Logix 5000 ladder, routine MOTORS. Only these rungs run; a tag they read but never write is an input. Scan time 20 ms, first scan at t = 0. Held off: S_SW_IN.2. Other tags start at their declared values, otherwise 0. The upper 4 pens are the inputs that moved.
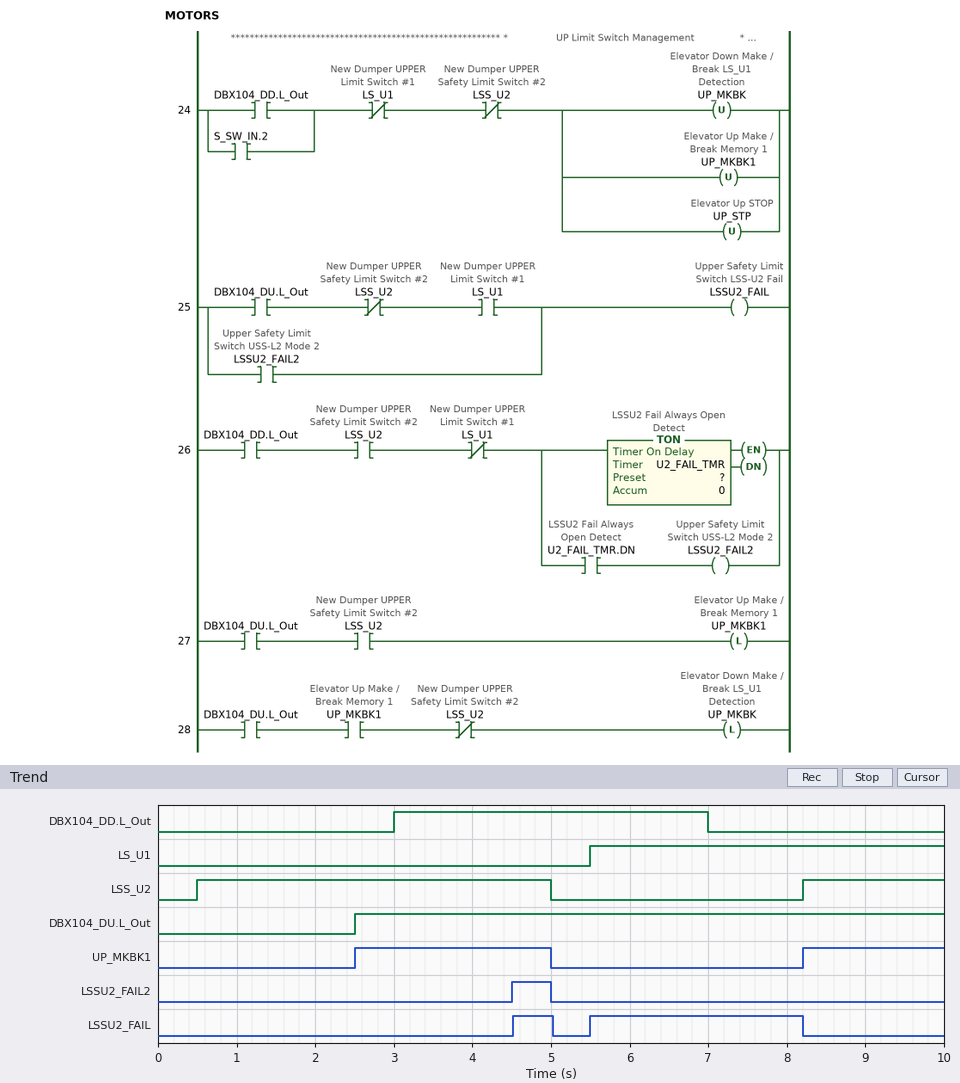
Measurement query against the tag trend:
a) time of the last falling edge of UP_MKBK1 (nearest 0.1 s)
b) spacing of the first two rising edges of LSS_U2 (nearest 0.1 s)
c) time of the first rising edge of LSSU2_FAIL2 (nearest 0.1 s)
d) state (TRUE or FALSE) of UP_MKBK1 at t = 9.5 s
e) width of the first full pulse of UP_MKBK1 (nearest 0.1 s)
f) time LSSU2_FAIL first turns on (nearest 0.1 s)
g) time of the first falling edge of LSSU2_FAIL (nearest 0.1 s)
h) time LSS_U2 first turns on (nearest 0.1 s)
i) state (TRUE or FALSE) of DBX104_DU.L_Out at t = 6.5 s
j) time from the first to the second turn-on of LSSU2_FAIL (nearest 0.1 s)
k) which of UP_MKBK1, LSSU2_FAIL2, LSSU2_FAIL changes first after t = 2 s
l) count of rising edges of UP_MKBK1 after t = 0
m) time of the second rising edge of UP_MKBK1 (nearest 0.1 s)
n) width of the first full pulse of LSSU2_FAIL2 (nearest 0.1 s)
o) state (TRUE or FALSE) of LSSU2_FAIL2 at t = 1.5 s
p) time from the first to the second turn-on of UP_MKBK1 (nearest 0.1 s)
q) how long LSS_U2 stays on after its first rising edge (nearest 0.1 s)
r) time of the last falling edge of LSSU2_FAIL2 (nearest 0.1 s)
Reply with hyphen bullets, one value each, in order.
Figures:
- 5.0 s
- 7.7 s
- 4.5 s
- TRUE
- 2.5 s
- 4.5 s
- 5.0 s
- 0.5 s
- TRUE
- 1.0 s
- UP_MKBK1
- 2
- 8.2 s
- 0.5 s
- FALSE
- 5.7 s
- 4.5 s
- 5.0 s
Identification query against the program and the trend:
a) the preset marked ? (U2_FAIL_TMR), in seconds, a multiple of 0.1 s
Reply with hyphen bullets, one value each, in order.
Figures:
- 1.5 s
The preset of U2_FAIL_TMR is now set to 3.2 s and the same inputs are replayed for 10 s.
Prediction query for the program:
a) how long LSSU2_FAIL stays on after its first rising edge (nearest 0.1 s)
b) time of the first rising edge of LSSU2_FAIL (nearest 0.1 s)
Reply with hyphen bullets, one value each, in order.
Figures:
- 2.7 s
- 5.5 s
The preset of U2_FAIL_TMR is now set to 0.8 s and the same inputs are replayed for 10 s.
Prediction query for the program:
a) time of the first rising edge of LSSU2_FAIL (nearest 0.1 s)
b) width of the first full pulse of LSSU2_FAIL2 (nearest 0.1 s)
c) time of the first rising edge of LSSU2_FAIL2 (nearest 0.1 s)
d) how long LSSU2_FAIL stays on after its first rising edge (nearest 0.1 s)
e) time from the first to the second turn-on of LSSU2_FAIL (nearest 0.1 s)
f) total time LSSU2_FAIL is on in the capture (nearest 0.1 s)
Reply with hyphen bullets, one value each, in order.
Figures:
- 3.8 s
- 1.2 s
- 3.8 s
- 1.2 s
- 1.7 s
- 3.9 s
